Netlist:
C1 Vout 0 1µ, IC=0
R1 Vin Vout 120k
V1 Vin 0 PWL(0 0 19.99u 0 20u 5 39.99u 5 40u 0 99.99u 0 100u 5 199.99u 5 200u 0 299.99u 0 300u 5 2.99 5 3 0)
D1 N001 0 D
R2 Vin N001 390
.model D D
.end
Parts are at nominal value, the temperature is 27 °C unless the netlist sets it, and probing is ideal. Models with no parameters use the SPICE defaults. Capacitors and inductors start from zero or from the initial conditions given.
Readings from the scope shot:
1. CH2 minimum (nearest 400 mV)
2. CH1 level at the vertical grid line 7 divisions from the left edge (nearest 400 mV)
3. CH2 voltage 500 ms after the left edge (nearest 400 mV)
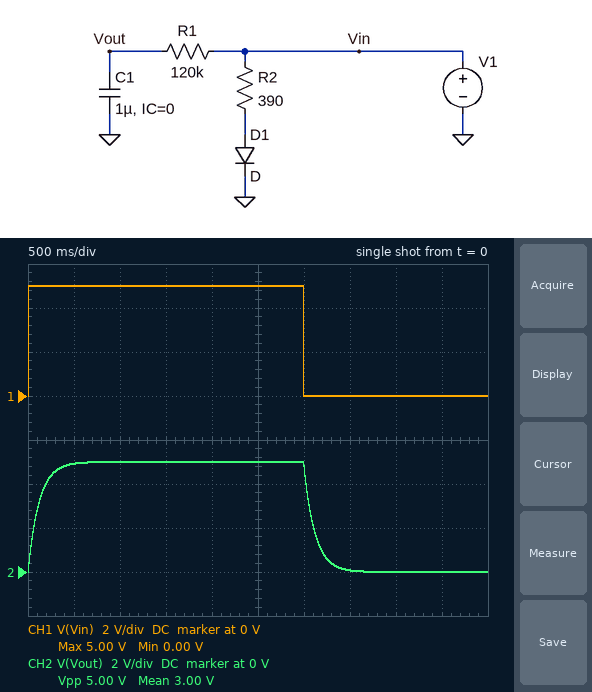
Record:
0 V
0 V
4.8 V
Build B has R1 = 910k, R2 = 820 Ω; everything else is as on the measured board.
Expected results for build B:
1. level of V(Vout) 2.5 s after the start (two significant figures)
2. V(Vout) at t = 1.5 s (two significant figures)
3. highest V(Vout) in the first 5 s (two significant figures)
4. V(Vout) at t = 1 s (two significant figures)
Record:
4.7 V
4.0 V
4.8 V
3.3 V
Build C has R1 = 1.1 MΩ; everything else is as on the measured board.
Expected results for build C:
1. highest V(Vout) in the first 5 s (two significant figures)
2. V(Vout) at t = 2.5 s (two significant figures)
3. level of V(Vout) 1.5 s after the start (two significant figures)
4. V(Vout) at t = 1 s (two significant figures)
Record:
4.7 V
4.5 V
3.7 V
3.0 V
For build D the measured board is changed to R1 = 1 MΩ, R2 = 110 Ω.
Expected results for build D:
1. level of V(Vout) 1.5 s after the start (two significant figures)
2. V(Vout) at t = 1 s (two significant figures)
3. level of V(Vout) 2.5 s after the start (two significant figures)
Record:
3.9 V
3.2 V
4.6 V
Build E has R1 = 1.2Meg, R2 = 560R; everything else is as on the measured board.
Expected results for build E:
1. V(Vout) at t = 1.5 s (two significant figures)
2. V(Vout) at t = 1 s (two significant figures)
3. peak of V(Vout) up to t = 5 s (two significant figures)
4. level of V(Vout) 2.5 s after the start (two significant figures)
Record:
3.6 V
2.8 V
4.6 V
4.4 V
